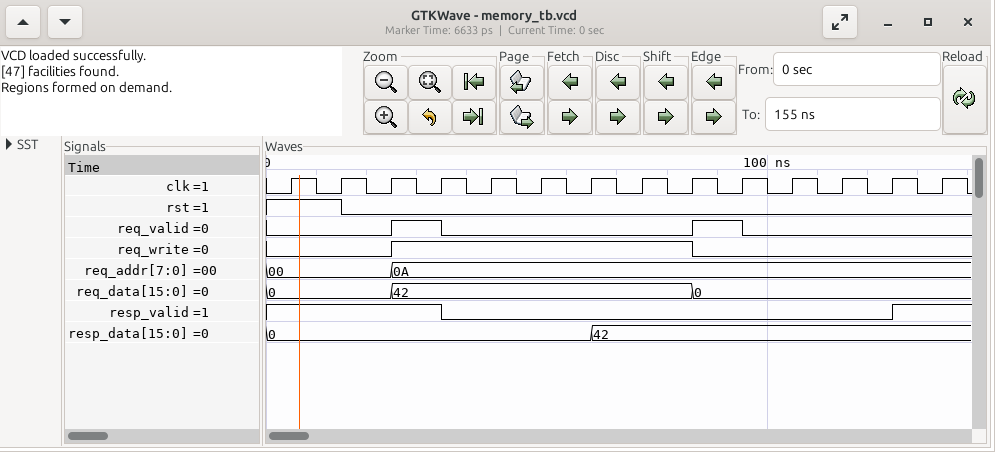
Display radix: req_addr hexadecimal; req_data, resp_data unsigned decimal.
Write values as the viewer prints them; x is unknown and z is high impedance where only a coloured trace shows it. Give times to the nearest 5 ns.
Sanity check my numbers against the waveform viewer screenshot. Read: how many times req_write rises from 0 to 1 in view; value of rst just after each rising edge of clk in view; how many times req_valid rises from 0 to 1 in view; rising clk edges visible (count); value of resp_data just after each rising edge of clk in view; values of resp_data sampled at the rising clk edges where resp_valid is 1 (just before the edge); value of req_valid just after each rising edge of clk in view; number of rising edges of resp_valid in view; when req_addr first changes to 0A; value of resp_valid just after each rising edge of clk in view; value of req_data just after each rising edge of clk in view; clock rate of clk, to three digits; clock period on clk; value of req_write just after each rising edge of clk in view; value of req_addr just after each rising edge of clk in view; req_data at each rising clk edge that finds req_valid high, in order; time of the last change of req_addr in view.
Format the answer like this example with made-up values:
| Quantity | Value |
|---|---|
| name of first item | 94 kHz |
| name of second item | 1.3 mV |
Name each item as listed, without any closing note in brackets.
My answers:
| Quantity | Value |
|---|---|
| how many times req_write rises from 0 to 1 in view | 1 |
| value of rst just after each rising edge of clk in view | 1 0 0 0 0 0 0 0 0 0 0 0 0 0 |
| how many times req_valid rises from 0 to 1 in view | 2 |
| rising clk edges visible | 14 |
| value of resp_data just after each rising edge of clk in view | 0, 0, 0, 0, 0, 0, 42, 42, 42, 42, 42, 42, 42, 42 |
| values of resp_data sampled at the rising clk edges where resp_valid is 1 | 0, 0, 0, 0, 42 |
| value of req_valid just after each rising edge of clk in view | 0 0 1 0 0 0 0 0 1 0 0 0 0 0 |
| number of rising edges of resp_valid in view | 1 |
| when req_addr first changes to 0A | 25 ns |
| value of resp_valid just after each rising edge of clk in view | 1 1 1 0 0 0 0 0 0 0 0 0 1 1 |
| value of req_data just after each rising edge of clk in view | 0, 0, 42, 42, 42, 42, 42, 42, 0, 0, 0, 0, 0, 0 |
| clock rate of clk, to three digits | 100 MHz |
| clock period on clk | 10 ns |
| value of req_write just after each rising edge of clk in view | 0 0 1 1 1 1 1 1 0 0 0 0 0 0 |
| value of req_addr just after each rising edge of clk in view | 00, 00, 0A, 0A, 0A, 0A, 0A, 0A, 0A, 0A, 0A, 0A, 0A, 0A |
| req_data at each rising clk edge that finds req_valid high, in order | 42, 0 |
| time of the last change of req_addr in view | 25 ns |
